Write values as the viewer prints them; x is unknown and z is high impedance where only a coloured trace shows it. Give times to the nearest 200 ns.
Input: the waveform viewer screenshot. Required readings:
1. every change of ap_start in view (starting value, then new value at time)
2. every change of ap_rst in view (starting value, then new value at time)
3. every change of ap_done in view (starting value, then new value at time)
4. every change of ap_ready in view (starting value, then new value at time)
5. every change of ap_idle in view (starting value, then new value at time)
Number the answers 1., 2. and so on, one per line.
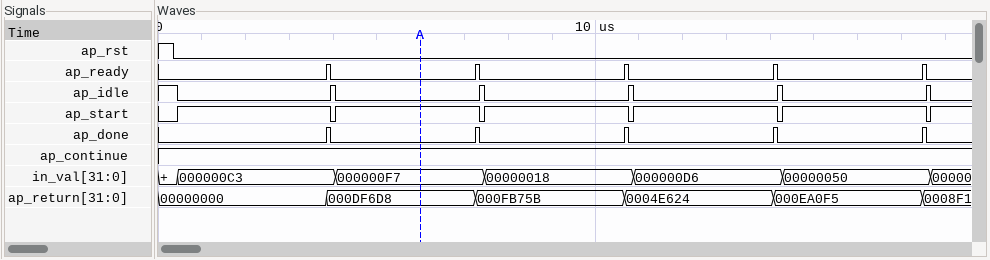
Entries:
1. 0, 1 at 400 ns, 0 at 4000 ns, 1 at 4000 ns, 0 at 7400 ns, 1 at 7400 ns, 0 at 10800 ns, 1 at 10800 ns, 0 at 14200 ns, 1 at 14200 ns, 0 at 17600 ns, 1 at 17600 ns
2. 1, 0 at 400 ns
3. 0, 1 at 3800 ns, 0 at 4000 ns, 1 at 7200 ns, 0 at 7400 ns, 1 at 10600 ns, 0 at 10800 ns, 1 at 14000 ns, 0 at 14200 ns, 1 at 17400 ns, 0 at 17600 ns
4. 0, 1 at 3800 ns, 0 at 4000 ns, 1 at 7200 ns, 0 at 7400 ns, 1 at 10600 ns, 0 at 10800 ns, 1 at 14000 ns, 0 at 14200 ns, 1 at 17400 ns, 0 at 17600 ns
5. 1, 0 at 400 ns, 1 at 4000 ns, 0 at 4000 ns, 1 at 7400 ns, 0 at 7400 ns, 1 at 10800 ns, 0 at 10800 ns, 1 at 14200 ns, 0 at 14200 ns, 1 at 17600 ns, 0 at 17600 ns
